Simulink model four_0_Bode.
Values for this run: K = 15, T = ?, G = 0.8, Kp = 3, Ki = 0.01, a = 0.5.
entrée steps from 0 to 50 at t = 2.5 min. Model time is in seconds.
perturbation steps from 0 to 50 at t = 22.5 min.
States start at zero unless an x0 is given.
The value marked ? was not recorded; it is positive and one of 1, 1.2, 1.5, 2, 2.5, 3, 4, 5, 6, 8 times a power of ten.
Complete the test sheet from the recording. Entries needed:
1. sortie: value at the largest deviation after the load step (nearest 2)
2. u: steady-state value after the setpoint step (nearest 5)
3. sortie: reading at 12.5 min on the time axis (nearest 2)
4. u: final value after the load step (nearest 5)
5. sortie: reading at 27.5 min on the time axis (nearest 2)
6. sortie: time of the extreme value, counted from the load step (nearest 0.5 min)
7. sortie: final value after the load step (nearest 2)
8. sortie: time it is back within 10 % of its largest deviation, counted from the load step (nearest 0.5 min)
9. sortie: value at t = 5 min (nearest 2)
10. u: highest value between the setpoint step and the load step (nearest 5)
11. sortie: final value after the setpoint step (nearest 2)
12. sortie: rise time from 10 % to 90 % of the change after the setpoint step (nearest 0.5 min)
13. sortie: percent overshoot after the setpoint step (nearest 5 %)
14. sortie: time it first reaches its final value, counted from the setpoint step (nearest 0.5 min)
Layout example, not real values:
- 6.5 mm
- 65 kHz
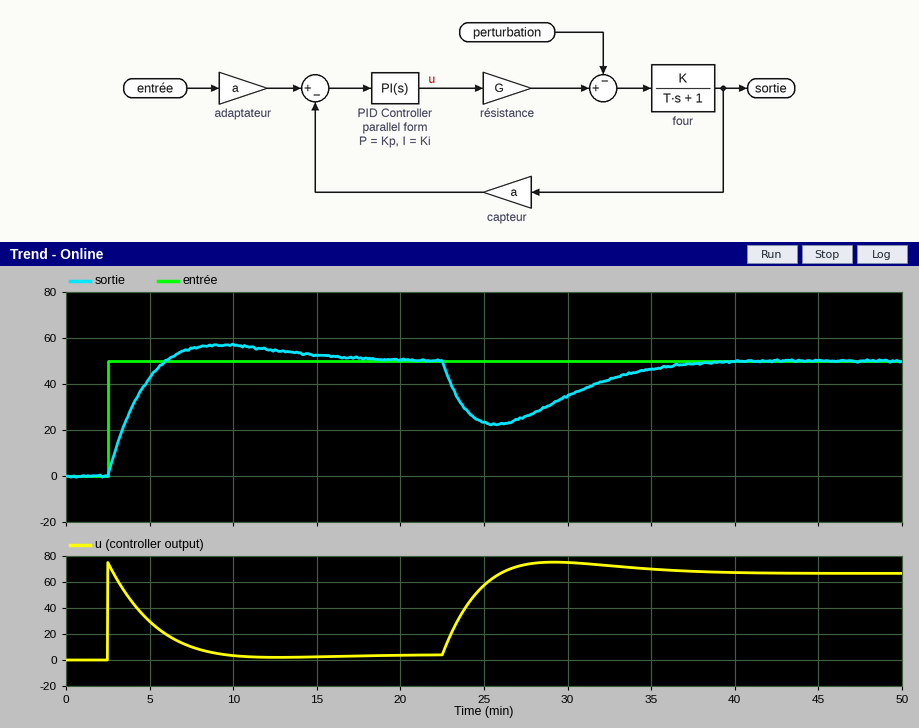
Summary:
- 22
- 5
- 54
- 65
- 26
- 3.0 min
- 50
- 13.0 min
- 42
- 75
- 50
- 2.5 min
- 15 %
- 3.5 min
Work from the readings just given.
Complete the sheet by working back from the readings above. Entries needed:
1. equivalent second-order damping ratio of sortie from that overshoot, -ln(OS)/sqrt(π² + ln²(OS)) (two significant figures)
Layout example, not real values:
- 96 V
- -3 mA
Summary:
- 0.52
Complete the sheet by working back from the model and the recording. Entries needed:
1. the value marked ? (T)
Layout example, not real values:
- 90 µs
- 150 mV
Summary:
- 2000
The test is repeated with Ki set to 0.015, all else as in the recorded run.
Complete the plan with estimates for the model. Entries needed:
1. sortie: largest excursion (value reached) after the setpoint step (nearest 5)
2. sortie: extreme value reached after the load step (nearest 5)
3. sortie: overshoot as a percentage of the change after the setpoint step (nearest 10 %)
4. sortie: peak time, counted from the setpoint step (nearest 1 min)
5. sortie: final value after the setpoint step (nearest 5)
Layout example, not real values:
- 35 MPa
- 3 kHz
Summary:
- 60
- 25
- 20 %
- 6 min
- 50
